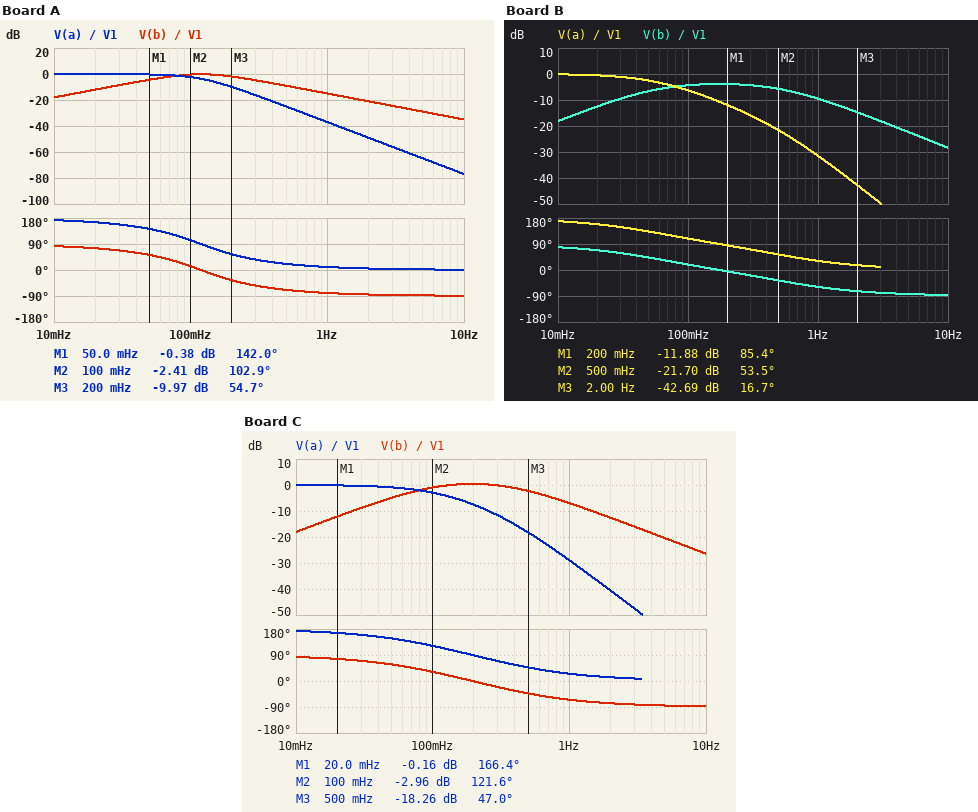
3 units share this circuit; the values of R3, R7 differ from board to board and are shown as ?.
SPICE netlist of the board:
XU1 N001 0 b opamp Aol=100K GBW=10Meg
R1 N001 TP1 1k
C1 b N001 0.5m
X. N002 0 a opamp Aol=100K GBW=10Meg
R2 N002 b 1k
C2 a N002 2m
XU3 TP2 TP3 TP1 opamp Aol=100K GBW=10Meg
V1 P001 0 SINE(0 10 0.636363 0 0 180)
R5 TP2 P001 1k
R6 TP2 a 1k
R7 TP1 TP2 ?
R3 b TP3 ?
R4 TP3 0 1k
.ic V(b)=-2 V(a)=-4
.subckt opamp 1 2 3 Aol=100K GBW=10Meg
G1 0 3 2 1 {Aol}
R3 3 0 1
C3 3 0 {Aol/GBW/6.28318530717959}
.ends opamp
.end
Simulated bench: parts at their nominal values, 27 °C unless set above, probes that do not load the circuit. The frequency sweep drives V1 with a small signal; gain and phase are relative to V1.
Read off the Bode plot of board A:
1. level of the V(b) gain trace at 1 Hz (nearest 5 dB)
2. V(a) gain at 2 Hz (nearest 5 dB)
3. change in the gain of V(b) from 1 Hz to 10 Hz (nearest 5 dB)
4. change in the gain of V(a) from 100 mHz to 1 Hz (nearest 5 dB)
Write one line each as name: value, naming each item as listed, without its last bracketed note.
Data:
level of the V(b) gain trace at 1 Hz: -15 dB
V(a) gain at 2 Hz: -50 dB
change in the gain of V(b) from 1 Hz to 10 Hz: -20 dB
change in the gain of V(a) from 100 mHz to 1 Hz: -35 dB
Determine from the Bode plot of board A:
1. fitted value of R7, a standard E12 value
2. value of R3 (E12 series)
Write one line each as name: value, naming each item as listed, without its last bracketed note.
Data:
fitted value of R7, a standard E12 value: 560 Ω
value of R3: 2.7 kΩ
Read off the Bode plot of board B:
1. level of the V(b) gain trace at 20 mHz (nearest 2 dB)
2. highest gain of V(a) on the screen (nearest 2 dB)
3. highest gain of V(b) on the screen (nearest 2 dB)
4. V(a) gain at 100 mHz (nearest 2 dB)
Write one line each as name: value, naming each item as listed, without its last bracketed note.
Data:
level of the V(b) gain trace at 20 mHz: -12 dB
highest gain of V(a) on the screen: 0 dB
highest gain of V(b) on the screen: -4 dB
V(a) gain at 100 mHz: -6 dB
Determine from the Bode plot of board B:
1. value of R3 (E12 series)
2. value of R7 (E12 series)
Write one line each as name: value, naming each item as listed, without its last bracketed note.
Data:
value of R3: 820 Ω
value of R7: 1.2 kΩ
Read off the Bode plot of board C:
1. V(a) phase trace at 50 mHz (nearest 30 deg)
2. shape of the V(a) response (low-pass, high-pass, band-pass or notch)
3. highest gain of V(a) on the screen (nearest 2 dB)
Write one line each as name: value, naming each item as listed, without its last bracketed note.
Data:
V(a) phase trace at 50 mHz: 150 deg
shape of the V(a) response: low-pass
highest gain of V(a) on the screen: 0 dB
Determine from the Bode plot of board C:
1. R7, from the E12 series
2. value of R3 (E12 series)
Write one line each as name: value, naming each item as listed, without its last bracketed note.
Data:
R7, from the E12 series: 1.5 kΩ
value of R3: 1.8 kΩ
